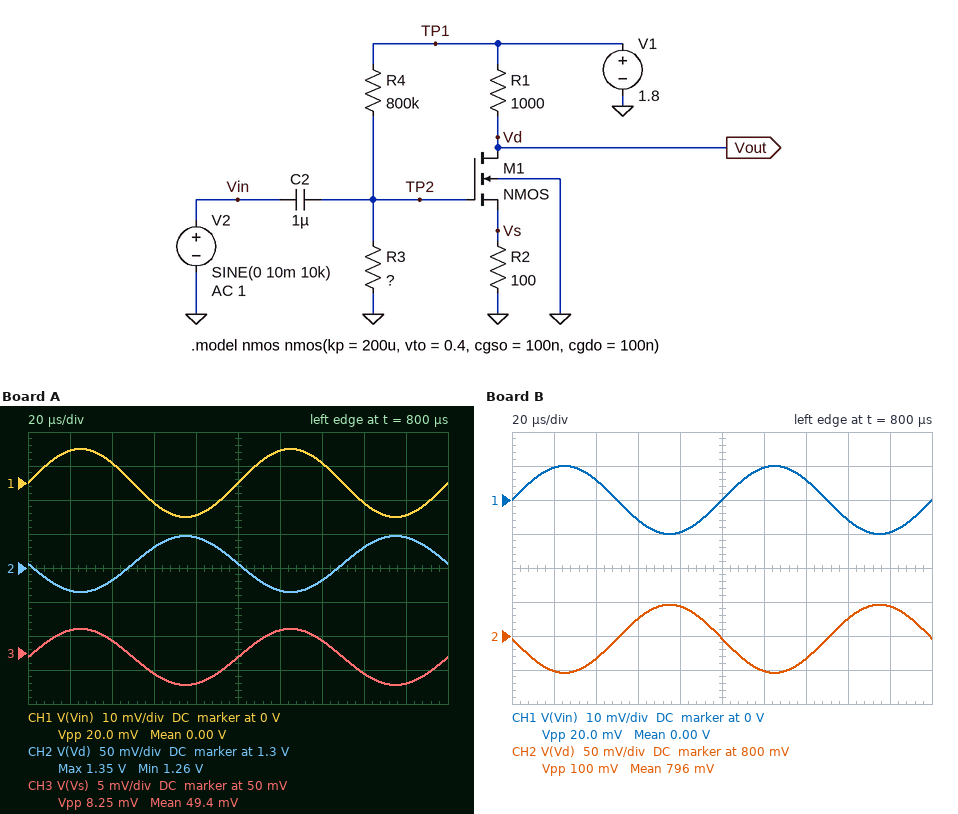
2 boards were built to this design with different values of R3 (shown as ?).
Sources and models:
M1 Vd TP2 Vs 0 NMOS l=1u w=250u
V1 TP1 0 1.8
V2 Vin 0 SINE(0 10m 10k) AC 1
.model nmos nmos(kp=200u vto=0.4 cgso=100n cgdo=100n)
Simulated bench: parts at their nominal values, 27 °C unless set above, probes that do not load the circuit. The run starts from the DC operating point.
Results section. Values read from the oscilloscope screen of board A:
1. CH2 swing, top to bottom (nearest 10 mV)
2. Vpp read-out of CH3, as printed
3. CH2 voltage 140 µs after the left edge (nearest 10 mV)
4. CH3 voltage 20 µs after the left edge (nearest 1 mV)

80 mV
8.25 mV
1.28 V
53 mV
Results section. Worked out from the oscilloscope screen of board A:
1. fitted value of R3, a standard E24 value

390 kΩ
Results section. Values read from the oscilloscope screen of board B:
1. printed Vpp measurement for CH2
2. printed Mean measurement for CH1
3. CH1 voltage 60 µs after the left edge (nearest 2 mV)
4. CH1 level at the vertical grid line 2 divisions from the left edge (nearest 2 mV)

100 mV
0.00 V
-6 mV
6 mV
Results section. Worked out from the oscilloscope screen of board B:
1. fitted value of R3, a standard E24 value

510 kΩ
